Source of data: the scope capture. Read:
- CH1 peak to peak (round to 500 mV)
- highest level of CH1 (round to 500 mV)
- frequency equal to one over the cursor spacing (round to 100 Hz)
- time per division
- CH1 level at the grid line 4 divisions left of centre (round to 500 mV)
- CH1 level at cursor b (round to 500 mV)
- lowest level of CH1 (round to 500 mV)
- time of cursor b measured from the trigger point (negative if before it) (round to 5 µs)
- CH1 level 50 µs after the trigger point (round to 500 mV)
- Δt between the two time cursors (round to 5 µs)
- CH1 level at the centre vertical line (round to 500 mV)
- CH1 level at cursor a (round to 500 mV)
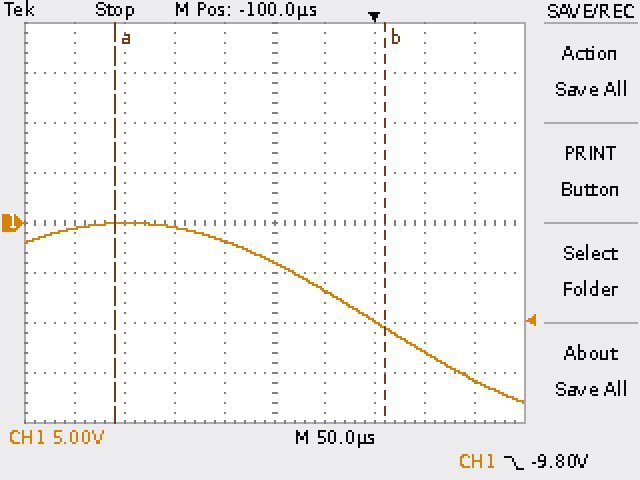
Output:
18.0 V
0.0 V
3.7 kHz
50 µs
-500 mV
-10.5 V
-18.0 V
+10 µs
-13.0 V
270 µs
-4.0 V
0.0 V
